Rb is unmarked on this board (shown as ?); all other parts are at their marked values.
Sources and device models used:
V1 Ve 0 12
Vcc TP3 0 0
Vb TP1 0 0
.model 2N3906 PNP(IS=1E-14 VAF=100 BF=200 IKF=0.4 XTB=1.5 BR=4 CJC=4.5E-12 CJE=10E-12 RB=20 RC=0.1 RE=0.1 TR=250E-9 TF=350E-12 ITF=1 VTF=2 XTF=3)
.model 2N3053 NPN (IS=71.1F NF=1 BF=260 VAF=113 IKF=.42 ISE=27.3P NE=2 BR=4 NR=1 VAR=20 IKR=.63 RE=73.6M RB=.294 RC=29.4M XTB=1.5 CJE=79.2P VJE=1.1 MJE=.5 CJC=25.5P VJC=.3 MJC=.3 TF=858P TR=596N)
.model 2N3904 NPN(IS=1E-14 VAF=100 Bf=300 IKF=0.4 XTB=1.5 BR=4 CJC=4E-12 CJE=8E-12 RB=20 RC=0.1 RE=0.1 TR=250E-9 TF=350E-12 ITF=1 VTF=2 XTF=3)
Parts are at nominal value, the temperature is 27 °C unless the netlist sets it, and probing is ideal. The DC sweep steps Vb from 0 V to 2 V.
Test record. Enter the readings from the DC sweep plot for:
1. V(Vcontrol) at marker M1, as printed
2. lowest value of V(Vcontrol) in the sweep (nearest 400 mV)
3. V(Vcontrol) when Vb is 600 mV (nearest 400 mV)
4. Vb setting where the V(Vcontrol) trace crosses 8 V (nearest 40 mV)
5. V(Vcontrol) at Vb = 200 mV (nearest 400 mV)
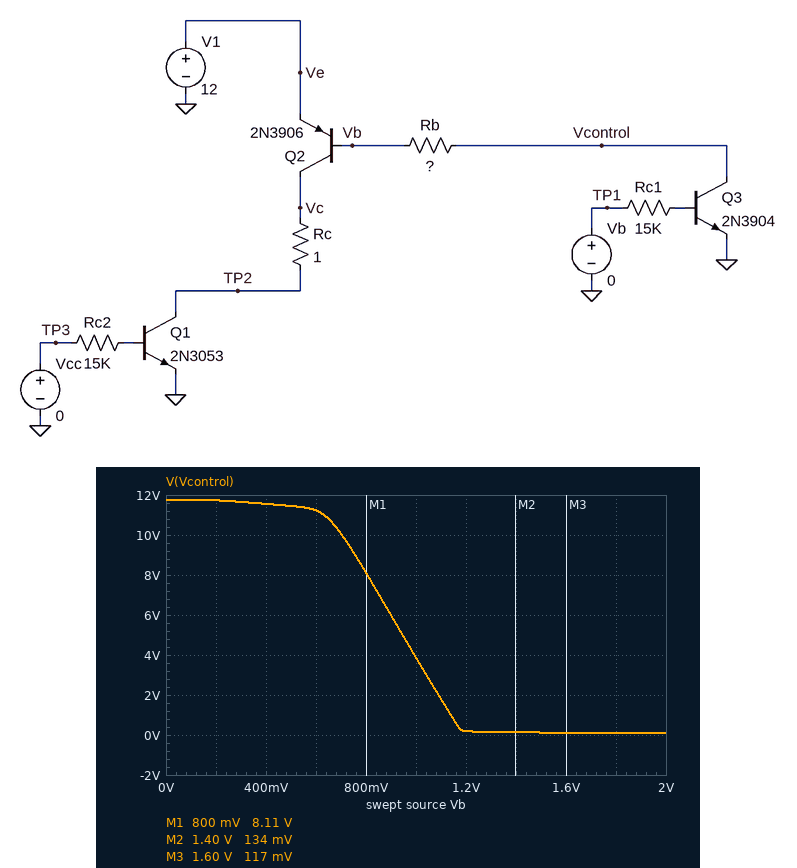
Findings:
8.11 V
0 V
11.2 V
800 mV
11.6 V
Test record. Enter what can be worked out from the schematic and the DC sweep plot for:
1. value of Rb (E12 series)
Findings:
1.2 kΩ
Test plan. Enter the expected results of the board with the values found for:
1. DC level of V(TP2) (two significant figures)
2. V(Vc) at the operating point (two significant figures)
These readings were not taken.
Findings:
12 V
12 V
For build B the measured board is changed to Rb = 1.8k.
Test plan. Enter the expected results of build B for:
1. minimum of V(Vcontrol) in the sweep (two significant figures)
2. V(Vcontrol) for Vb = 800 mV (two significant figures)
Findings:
85 mV
6.6 V
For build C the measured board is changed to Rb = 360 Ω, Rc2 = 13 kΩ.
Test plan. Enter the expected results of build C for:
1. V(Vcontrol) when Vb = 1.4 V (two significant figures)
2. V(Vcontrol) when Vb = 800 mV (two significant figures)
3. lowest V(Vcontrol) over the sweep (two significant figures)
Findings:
6.0 V
10 V
2.1 V
